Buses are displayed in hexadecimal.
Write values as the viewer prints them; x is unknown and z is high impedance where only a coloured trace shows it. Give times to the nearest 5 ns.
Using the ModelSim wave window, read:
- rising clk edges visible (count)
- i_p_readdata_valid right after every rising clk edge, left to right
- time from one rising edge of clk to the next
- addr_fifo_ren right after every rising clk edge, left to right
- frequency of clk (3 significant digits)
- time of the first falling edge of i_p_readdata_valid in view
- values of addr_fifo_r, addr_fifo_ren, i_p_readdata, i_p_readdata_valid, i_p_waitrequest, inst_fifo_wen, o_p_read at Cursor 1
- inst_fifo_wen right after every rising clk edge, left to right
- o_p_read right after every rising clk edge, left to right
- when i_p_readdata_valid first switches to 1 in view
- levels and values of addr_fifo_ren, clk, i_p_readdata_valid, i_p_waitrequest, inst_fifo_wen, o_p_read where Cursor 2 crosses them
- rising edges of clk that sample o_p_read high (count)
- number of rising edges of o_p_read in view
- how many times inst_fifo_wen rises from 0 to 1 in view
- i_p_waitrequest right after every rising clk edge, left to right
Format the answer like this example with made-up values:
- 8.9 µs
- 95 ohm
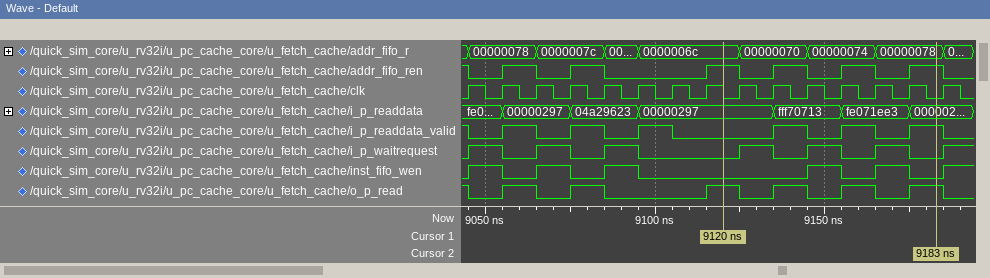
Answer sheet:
- 15
- 0 1 0 1 0 1 0 0 0 1 0 1 0 1 0
- 10 ns
- 0 1 0 1 0 0 0 1 0 1 0 1 0 1 0
- 100 MHz
- 9045 ns
- addr_fifo_r=0000006c, addr_fifo_ren=1, i_p_readdata=00000297, i_p_readdata_valid=0, i_p_waitrequest=0, inst_fifo_wen=0, o_p_read=1
- 1 0 1 0 1 0 0 0 0 0 1 0 1 0 1
- 0 1 0 1 0 0 0 1 0 1 0 1 0 1 0
- 9055 ns
- addr_fifo_ren=1, clk=0, i_p_readdata_valid=1, i_p_waitrequest=0, inst_fifo_wen=0, o_p_read=1
- 7
- 6
- 6
- 1 0 1 0 1 0 0 0 1 0 1 0 1 0 1
